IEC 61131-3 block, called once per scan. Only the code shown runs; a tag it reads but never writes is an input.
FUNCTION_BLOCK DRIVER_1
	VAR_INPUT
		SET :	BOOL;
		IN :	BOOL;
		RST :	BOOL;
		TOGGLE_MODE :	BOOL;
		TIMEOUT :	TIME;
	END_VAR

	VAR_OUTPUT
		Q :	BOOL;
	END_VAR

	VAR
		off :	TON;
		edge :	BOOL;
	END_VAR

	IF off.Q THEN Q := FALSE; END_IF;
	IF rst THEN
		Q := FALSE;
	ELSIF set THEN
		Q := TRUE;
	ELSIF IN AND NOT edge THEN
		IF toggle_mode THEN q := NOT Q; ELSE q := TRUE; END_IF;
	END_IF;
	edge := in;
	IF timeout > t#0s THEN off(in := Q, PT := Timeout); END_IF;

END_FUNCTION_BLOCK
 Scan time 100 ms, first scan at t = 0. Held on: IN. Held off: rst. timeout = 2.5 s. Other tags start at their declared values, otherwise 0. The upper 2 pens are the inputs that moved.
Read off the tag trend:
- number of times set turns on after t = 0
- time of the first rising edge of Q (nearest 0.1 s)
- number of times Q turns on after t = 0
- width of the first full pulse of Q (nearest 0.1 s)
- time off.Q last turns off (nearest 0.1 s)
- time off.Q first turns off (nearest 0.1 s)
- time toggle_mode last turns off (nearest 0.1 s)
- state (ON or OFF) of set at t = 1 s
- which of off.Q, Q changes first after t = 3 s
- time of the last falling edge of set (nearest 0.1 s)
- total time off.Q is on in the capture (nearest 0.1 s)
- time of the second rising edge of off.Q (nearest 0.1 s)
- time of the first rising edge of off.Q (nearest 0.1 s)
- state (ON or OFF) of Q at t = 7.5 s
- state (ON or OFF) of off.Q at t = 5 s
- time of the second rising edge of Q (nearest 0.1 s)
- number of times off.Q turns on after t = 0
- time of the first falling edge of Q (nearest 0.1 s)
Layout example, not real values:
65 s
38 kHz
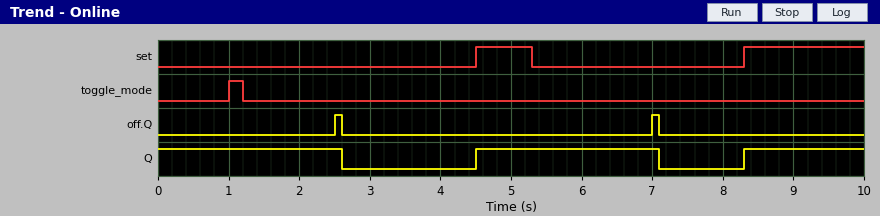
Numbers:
2
4.5 s
2
2.6 s
7.1 s
2.6 s
1.2 s
OFF
Q
5.3 s
0.2 s
7.0 s
2.5 s
OFF
OFF
8.3 s
2
2.6 s
